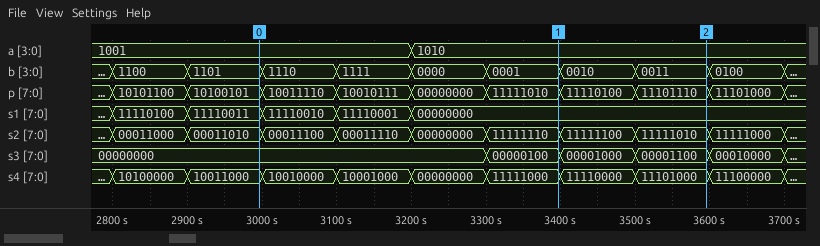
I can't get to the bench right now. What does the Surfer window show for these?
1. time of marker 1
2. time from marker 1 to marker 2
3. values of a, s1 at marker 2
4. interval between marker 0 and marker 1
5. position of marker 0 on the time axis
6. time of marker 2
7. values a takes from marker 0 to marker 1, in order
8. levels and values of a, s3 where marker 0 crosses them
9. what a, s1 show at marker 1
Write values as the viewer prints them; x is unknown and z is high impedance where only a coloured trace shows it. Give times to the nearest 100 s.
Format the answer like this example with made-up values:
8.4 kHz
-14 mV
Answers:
3400 s
200 s
a=1010, s1=00000000
400 s
3000 s
3600 s
1001, 1010
a=1001, s3=00000000
a=1010, s1=00000000
